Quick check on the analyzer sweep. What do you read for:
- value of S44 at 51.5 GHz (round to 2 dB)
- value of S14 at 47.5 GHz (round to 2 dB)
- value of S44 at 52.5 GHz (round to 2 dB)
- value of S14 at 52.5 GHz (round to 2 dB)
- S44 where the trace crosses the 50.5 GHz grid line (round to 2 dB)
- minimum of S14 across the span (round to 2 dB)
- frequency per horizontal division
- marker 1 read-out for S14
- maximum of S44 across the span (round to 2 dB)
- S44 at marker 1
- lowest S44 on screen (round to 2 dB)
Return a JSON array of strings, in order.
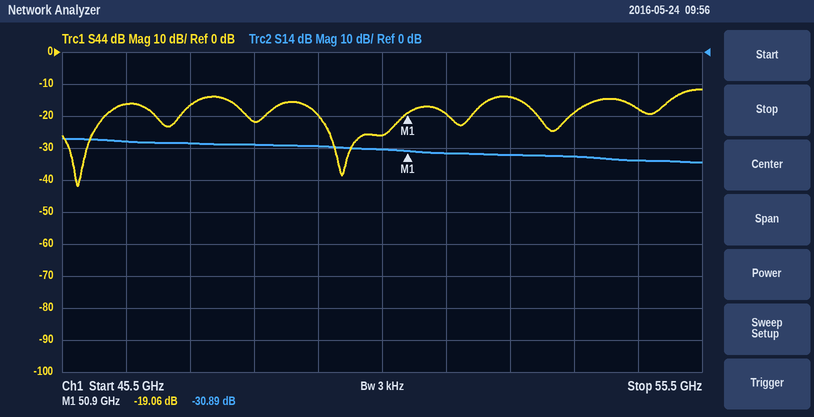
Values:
["-20 dB", "-28 dB", "-14 dB", "-32 dB", "-26 dB", "-34 dB", "1 GHz", "-30.89 dB", "-12 dB", "-19.06 dB", "-42 dB"]
